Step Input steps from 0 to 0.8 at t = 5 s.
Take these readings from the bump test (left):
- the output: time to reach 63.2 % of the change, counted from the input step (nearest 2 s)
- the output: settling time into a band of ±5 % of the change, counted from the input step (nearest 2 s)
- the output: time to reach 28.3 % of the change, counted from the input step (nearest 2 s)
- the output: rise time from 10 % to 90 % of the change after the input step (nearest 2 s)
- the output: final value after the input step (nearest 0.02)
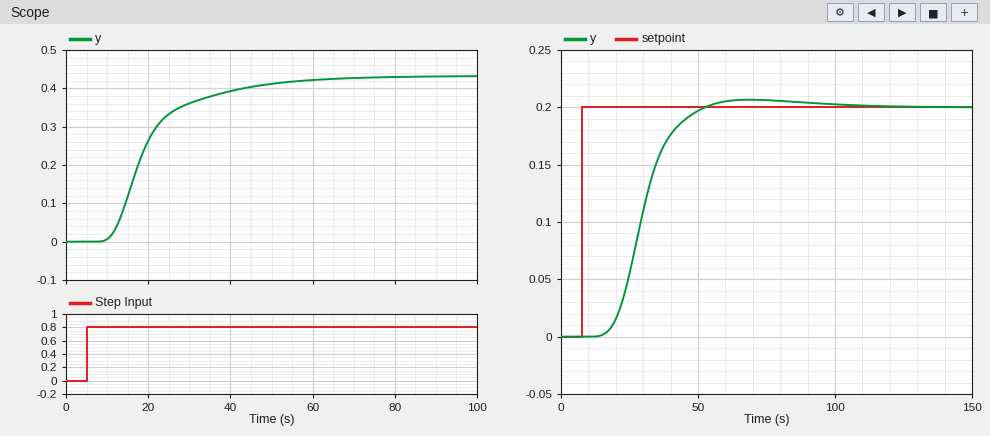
16 s
44 s
10 s
26 s
0.44
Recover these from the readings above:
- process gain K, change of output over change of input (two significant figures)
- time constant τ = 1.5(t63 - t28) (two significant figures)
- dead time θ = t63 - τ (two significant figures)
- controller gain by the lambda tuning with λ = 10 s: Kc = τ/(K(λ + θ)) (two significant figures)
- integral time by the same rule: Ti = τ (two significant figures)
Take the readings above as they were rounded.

0.55
9.0 s
7.0 s
0.96
9.0 s
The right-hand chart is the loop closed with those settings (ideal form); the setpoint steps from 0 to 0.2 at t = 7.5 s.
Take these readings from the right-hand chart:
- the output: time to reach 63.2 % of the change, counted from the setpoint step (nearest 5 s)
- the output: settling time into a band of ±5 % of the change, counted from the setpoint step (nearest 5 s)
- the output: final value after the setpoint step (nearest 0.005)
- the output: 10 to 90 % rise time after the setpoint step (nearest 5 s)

25 s
40 s
0.200
20 s
